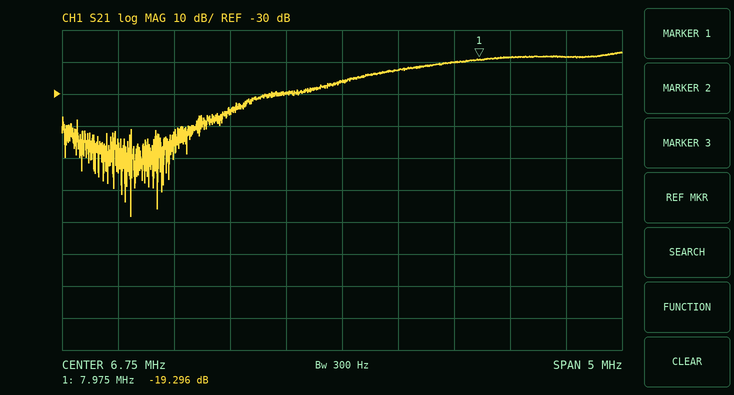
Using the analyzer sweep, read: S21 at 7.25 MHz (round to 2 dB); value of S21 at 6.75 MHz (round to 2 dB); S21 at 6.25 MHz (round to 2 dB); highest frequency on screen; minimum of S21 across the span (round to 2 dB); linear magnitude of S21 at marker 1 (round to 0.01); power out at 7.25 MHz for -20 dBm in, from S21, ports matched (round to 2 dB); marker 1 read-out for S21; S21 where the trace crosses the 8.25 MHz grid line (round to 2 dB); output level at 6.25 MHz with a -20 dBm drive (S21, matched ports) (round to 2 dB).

-22 dB
-26 dB
-30 dB
9.25 MHz
-68 dB
0.11
-42 dBm
-19.296 dB
-18 dB
-50 dBm
